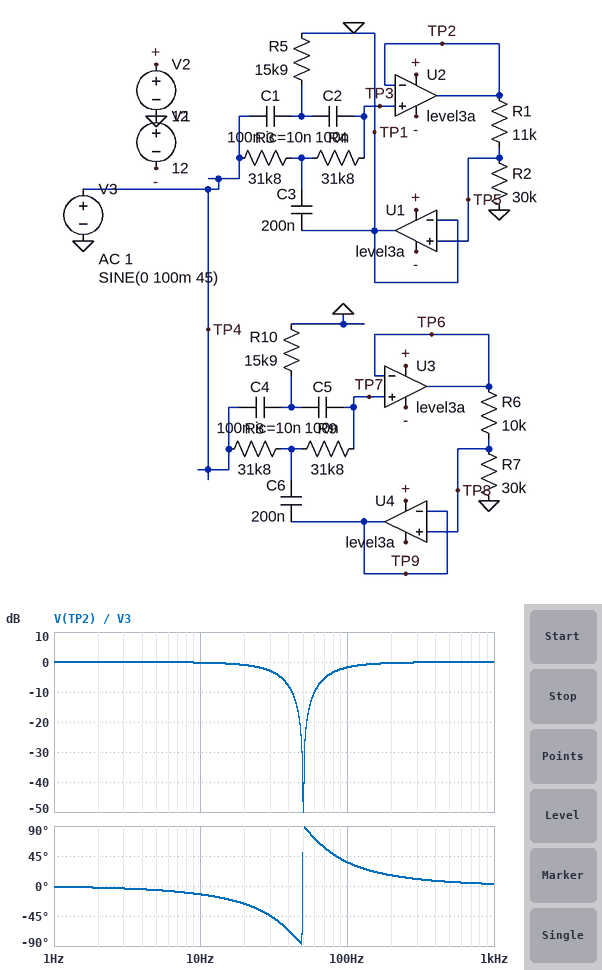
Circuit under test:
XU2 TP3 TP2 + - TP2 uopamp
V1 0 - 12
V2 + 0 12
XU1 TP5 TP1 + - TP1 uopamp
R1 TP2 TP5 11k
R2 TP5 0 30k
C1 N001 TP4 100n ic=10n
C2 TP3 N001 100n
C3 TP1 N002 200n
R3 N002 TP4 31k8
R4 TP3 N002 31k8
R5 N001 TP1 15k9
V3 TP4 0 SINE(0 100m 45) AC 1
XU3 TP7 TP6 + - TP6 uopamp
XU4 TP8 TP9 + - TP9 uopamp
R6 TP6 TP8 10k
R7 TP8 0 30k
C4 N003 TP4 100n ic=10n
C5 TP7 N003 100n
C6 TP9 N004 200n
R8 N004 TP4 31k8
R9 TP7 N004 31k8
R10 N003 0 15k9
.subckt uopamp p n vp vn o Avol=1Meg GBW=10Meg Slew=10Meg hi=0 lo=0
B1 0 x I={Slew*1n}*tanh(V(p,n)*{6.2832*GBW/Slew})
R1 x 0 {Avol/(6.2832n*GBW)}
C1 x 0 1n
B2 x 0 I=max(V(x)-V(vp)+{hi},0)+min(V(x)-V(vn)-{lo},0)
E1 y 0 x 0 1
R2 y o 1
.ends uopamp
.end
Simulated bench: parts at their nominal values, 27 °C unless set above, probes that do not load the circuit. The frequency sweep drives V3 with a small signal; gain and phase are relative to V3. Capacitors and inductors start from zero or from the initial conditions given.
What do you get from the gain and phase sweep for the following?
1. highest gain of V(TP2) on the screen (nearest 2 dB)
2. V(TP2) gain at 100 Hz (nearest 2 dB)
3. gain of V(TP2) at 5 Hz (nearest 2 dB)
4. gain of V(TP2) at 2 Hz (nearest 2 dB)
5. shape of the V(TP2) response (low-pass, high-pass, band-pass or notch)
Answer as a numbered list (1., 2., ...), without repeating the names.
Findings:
1. 0 dB
2. -2 dB
3. 0 dB
4. 0 dB
5. notch
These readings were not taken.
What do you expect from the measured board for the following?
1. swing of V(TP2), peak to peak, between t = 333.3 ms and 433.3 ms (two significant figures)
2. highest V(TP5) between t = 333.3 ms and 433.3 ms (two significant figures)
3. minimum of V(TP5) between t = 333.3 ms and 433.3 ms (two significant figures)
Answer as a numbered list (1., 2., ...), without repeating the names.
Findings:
1. 39 mV
2. 14 mV
3. -14 mV
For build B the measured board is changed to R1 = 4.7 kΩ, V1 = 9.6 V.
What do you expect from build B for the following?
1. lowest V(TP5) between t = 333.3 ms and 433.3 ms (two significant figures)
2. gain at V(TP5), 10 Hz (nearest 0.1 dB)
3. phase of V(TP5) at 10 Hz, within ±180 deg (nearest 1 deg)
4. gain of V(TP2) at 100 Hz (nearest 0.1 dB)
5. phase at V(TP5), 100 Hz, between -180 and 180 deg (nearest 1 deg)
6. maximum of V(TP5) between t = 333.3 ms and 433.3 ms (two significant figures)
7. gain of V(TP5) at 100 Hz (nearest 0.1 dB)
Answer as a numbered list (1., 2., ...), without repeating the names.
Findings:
1. -32 mV
2. -1.3 dB
3. -6 deg
4. -0.5 dB
5. 20 deg
6. 32 mV
7. -1.8 dB
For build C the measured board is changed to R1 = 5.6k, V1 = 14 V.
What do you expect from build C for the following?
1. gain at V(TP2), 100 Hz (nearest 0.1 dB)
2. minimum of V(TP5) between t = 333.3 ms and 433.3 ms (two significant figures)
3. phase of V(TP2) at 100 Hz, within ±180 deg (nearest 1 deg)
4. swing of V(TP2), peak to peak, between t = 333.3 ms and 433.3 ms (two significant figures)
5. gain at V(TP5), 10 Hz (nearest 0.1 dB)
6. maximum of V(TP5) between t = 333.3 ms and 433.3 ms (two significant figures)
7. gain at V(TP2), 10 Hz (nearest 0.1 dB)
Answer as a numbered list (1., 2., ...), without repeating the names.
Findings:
1. -0.7 dB
2. -27 mV
3. 23 deg
4. 64 mV
5. -1.6 dB
6. 27 mV
7. -0.1 dB
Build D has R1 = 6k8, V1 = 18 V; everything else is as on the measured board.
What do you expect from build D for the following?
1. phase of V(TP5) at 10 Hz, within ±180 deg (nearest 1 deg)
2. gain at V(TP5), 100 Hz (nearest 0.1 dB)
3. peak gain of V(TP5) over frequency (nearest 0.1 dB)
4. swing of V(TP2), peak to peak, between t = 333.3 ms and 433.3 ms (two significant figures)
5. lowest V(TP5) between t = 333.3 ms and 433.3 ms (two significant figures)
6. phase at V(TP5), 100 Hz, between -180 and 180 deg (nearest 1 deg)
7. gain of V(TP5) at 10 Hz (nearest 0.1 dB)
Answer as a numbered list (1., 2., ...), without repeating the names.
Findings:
1. -9 deg
2. -2.7 dB
3. -1.8 dB
4. 55 mV
5. -23 mV
6. 26 deg
7. -1.9 dB
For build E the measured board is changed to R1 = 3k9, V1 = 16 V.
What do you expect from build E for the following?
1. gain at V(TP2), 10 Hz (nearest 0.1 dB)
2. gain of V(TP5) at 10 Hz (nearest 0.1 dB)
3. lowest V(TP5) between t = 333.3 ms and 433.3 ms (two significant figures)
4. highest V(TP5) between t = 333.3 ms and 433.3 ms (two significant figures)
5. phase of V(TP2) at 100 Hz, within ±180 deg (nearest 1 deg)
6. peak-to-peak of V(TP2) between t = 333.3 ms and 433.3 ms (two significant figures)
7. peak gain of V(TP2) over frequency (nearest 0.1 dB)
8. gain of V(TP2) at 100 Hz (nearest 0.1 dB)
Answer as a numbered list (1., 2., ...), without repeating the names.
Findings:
1. 0 dB
2. -1.1 dB
3. -37 mV
4. 37 mV
5. 17 deg
6. 84 mV
7. 0 dB
8. -0.4 dB
